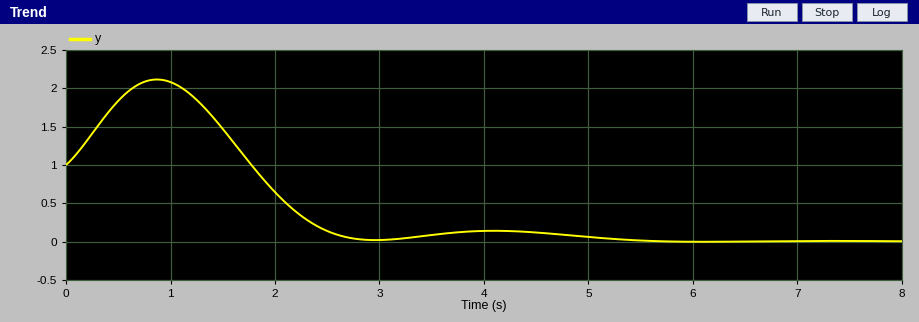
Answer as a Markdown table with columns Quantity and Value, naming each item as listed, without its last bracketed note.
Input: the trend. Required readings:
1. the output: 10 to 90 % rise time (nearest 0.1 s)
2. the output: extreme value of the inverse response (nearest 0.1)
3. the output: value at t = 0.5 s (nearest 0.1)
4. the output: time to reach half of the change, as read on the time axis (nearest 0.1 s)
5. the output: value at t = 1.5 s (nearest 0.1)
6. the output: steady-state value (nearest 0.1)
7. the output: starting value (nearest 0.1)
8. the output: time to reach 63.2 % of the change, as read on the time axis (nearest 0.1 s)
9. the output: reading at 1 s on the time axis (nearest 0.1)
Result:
| Quantity | Value |
|---|---|
| the output: 10 to 90 % rise time | 0.7 s |
| the output: extreme value of the inverse response | 2.1 |
| the output: value at t = 0.5 s | 1.8 |
| the output: time to reach half of the change, as read on the time axis | 2.1 s |
| the output: value at t = 1.5 s | 1.5 |
| the output: steady-state value | 0.0 |
| the output: starting value | 1.0 |
| the output: time to reach 63.2 % of the change, as read on the time axis | 2.2 s |
| the output: reading at 1 s on the time axis | 2.1 |
